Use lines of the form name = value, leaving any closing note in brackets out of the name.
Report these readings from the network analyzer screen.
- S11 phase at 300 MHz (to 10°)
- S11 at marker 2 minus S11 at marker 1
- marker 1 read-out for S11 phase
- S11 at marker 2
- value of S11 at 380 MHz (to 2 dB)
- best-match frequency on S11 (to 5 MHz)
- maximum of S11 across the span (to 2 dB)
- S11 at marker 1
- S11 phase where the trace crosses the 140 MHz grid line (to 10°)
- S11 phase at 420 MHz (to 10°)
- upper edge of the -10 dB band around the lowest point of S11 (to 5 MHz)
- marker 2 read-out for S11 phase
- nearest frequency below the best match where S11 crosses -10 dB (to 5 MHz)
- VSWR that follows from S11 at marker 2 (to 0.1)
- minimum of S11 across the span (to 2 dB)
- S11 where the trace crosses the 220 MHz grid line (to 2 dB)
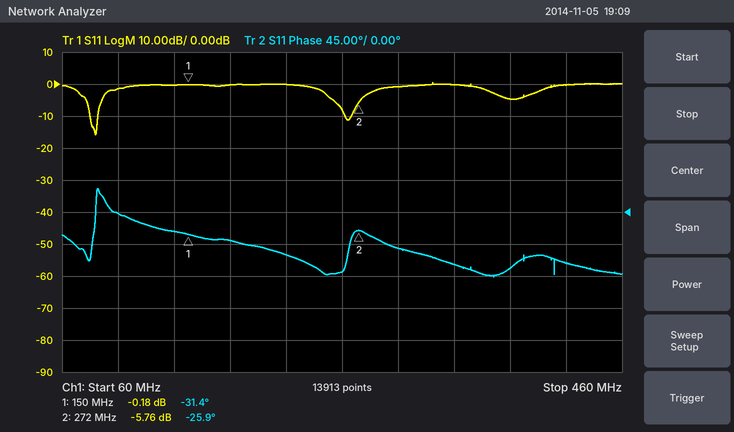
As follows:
S11 phase at 300 MHz = -50°
S11 at marker 2 minus S11 at marker 1 = -5.58 dB
marker 1 read-out for S11 phase = -31.4°
S11 at marker 2 = -5.76 dB
value of S11 at 380 MHz = -4 dB
best-match frequency on S11 = 85 MHz
maximum of S11 across the span = 0 dB
S11 at marker 1 = -0.18 dB
S11 phase where the trace crosses the 140 MHz grid line = -30°
S11 phase at 420 MHz = -70°
upper edge of the -10 dB band around the lowest point of S11 = 85 MHz
marker 2 read-out for S11 phase = -25.9°
nearest frequency below the best match where S11 crosses -10 dB = 80 MHz
VSWR that follows from S11 at marker 2 = 3.1
minimum of S11 across the span = -16 dB
S11 where the trace crosses the 220 MHz grid line = 0 dB
